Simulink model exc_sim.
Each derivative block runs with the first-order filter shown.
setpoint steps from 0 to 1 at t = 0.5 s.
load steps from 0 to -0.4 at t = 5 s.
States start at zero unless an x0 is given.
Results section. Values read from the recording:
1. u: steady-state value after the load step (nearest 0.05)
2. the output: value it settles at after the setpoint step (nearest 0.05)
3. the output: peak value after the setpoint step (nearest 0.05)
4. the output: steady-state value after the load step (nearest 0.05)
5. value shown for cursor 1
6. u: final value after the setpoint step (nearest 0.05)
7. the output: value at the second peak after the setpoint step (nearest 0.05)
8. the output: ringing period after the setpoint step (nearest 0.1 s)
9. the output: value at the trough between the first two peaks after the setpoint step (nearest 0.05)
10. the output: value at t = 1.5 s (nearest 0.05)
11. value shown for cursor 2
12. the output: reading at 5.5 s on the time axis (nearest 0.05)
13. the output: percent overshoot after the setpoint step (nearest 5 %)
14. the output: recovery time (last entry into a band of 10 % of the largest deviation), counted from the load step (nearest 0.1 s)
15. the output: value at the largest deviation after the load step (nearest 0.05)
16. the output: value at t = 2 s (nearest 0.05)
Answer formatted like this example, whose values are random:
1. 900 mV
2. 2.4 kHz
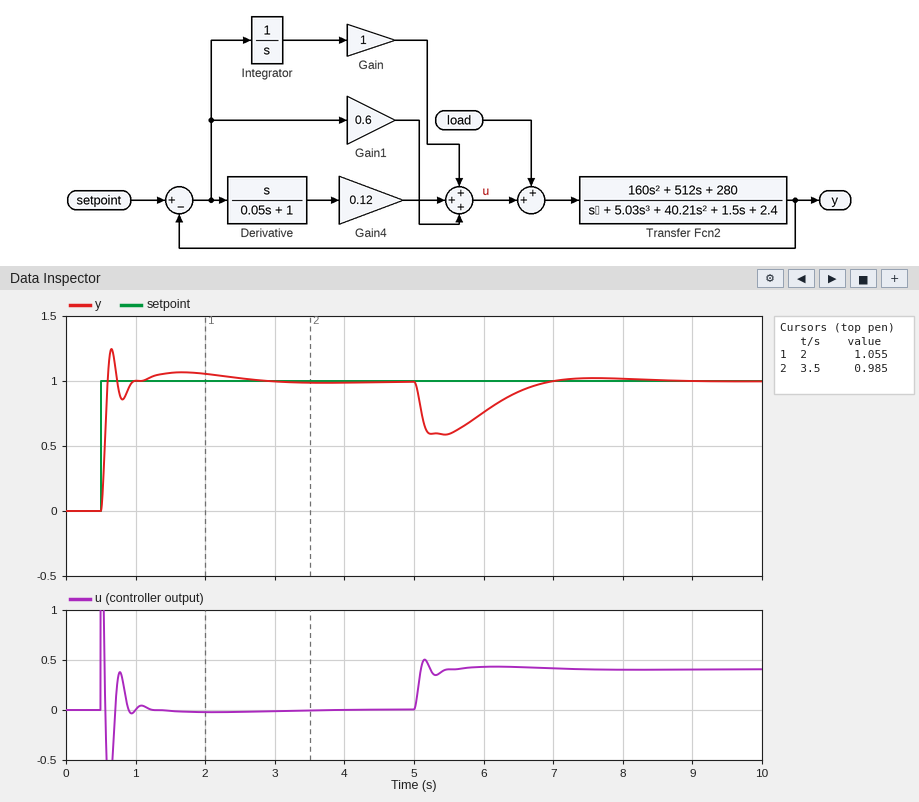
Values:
1. 0.40
2. 1.00
3. 1.25
4. 1.00
5. 1.055
6. 0.00
7. 1.05
8. 1.0 s
9. 0.85
10. 1.05
11. 0.985
12. 0.60
13. 25 %
14. 1.7 s
15. 0.60
16. 1.05
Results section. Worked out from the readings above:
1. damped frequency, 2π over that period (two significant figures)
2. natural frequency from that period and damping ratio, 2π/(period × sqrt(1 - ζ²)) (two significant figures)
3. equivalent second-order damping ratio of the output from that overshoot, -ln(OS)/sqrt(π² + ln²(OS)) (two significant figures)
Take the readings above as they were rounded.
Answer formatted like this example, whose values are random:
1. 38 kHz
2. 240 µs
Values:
1. 6.3 rad/s
2. 6.9 rad/s
3. 0.40
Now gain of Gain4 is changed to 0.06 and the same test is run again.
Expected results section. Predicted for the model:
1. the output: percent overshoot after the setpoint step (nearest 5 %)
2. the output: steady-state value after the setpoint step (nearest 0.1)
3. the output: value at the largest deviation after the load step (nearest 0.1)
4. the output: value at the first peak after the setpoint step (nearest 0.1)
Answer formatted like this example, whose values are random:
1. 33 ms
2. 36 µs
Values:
1. 30 %
2. 1.0
3. 0.4
4. 1.3
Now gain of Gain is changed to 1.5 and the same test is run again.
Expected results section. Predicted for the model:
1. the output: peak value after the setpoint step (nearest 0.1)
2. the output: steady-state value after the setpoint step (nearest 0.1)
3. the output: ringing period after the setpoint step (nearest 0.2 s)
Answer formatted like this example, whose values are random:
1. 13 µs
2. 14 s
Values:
1. 1.3
2. 1.0
3. 0.8 s
